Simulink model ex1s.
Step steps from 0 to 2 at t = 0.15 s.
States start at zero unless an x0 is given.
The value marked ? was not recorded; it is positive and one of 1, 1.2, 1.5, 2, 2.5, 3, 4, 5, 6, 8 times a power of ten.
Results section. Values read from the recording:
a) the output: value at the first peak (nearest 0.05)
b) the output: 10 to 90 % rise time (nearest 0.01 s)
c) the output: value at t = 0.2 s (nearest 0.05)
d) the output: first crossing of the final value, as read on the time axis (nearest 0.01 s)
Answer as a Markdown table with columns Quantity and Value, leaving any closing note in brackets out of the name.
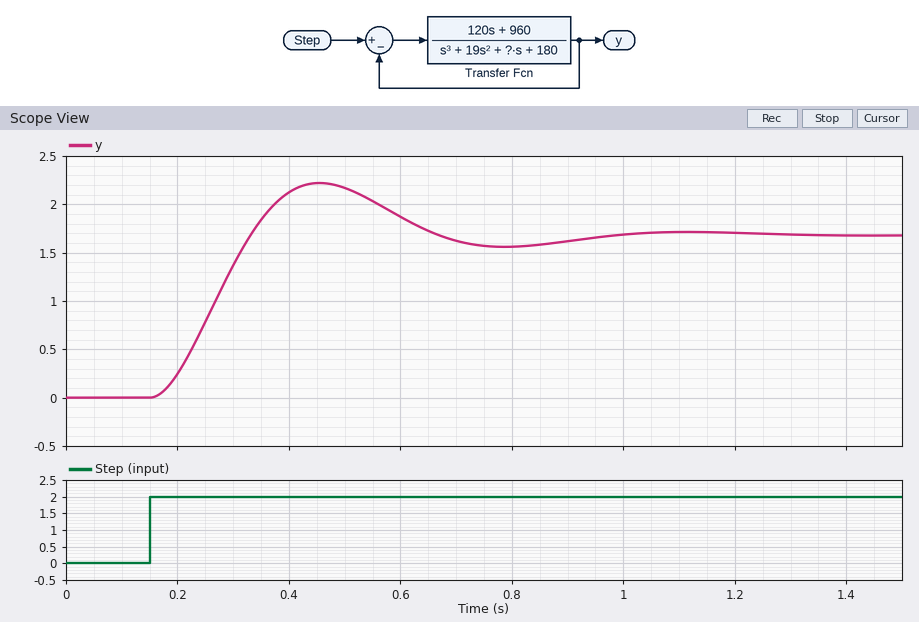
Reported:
| Quantity | Value |
|---|---|
| the output: value at the first peak | 2.20 |
| the output: 10 to 90 % rise time | 0.12 s |
| the output: value at t = 0.2 s | 0.25 |
| the output: first crossing of the final value, as read on the time axis | 0.33 s |
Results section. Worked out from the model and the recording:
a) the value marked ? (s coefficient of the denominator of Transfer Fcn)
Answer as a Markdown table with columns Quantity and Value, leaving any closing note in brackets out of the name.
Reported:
| Quantity | Value |
|---|---|
| the value marked ? | 80 |
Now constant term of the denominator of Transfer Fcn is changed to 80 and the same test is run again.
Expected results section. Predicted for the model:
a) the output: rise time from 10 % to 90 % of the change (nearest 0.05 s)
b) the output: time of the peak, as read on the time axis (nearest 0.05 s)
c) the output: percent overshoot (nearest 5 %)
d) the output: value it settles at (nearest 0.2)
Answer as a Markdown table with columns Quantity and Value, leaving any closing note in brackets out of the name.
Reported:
| Quantity | Value |
|---|---|
| the output: rise time from 10 % to 90 % of the change | 0.15 s |
| the output: time of the peak, as read on the time axis | 0.45 s |
| the output: percent overshoot | 25 % |
| the output: value it settles at | 1.8 |
